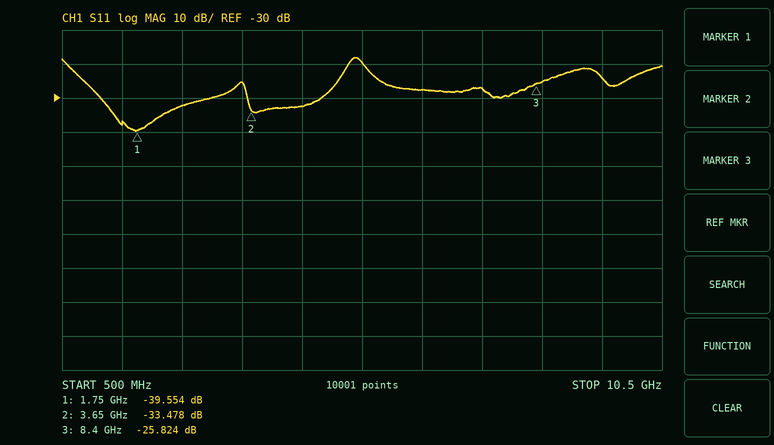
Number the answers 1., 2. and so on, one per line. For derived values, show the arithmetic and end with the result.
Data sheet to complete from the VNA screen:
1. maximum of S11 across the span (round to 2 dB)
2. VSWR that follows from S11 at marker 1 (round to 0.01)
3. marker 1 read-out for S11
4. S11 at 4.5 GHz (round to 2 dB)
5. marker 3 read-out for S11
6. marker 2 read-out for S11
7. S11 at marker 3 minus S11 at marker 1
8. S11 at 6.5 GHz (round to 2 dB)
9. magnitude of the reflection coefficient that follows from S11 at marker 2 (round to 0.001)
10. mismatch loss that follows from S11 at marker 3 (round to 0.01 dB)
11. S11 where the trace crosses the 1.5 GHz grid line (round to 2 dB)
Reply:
1. -18 dB
2. (1 + 0.0105)/(1 − 0.0105) ≈ 1.02
3. -39.554 dB
4. -32 dB
5. -25.824 dB
6. -33.478 dB
7. -25.824 − (-39.554) = 13.730 dB
8. -28 dB
9. 10^(-33.478/20) ≈ 0.021
10. −10 log10(1 − 10^(-25.824/10)) ≈ 0.01 dB
11. -38 dB
